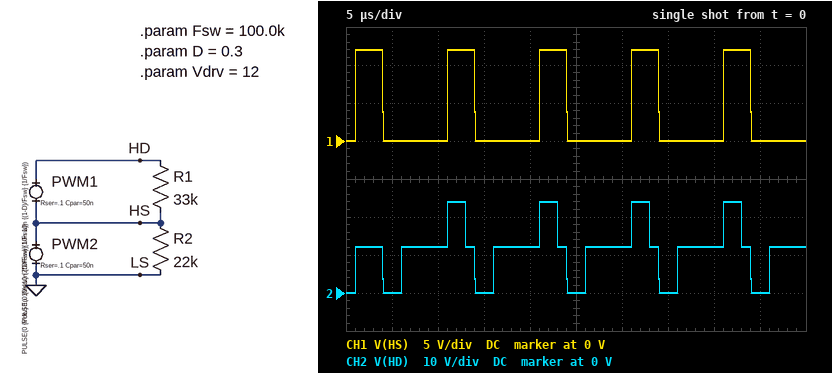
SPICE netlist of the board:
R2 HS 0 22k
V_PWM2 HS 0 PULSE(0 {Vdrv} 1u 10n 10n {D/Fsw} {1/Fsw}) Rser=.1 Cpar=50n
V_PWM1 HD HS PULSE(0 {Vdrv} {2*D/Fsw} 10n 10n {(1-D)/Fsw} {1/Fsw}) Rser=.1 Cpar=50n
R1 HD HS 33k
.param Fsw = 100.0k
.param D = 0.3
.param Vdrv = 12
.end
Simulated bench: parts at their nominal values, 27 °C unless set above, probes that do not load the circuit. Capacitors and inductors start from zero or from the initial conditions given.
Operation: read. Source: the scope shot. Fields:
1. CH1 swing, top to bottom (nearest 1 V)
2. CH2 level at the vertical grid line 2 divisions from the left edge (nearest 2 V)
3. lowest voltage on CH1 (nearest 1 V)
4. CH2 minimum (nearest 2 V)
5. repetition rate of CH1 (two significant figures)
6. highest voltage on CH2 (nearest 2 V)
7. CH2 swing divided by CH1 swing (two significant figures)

12 V
12 V
0 V
0 V
100 kHz
24 V
2.0
